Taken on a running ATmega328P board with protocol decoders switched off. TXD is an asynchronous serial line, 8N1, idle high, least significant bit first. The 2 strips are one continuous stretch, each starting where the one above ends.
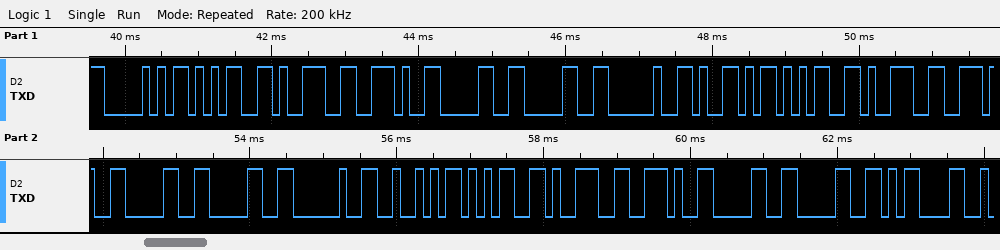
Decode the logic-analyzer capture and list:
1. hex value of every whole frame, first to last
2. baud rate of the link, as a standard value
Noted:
50 35 39 2E 30 30 20 59 35 39 2E 30 30 20 52 35 39 2E 30 30 0D
9600 baud
